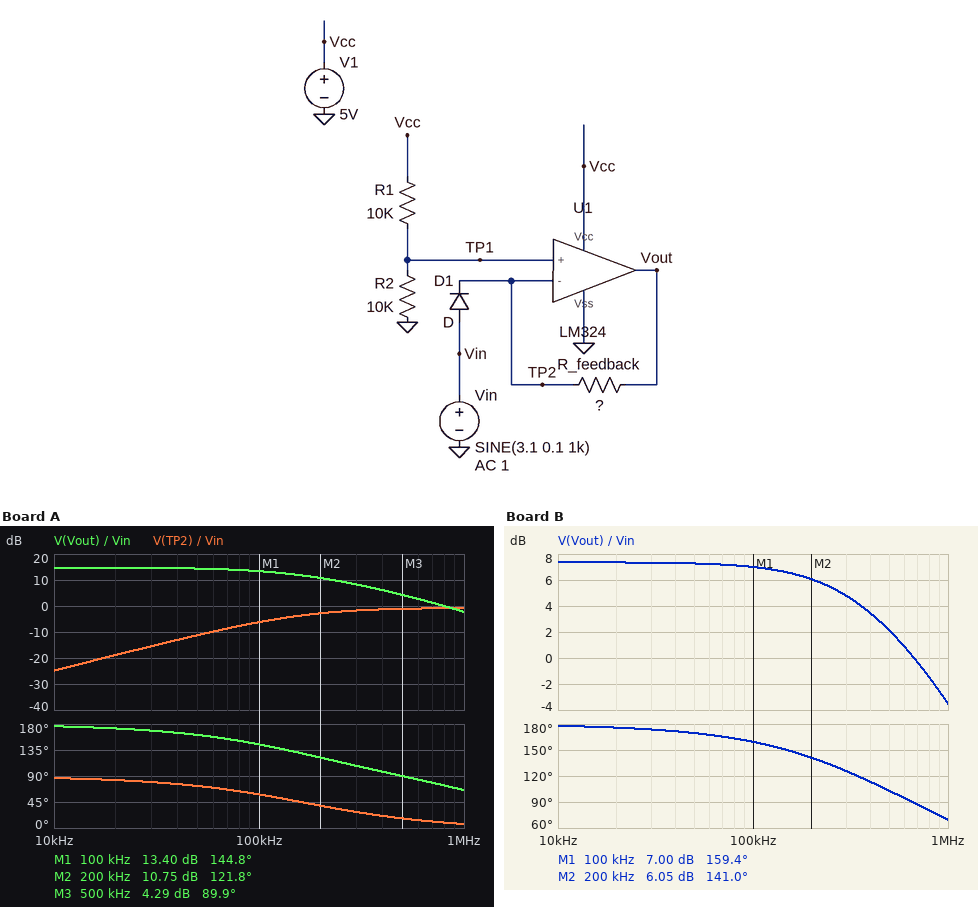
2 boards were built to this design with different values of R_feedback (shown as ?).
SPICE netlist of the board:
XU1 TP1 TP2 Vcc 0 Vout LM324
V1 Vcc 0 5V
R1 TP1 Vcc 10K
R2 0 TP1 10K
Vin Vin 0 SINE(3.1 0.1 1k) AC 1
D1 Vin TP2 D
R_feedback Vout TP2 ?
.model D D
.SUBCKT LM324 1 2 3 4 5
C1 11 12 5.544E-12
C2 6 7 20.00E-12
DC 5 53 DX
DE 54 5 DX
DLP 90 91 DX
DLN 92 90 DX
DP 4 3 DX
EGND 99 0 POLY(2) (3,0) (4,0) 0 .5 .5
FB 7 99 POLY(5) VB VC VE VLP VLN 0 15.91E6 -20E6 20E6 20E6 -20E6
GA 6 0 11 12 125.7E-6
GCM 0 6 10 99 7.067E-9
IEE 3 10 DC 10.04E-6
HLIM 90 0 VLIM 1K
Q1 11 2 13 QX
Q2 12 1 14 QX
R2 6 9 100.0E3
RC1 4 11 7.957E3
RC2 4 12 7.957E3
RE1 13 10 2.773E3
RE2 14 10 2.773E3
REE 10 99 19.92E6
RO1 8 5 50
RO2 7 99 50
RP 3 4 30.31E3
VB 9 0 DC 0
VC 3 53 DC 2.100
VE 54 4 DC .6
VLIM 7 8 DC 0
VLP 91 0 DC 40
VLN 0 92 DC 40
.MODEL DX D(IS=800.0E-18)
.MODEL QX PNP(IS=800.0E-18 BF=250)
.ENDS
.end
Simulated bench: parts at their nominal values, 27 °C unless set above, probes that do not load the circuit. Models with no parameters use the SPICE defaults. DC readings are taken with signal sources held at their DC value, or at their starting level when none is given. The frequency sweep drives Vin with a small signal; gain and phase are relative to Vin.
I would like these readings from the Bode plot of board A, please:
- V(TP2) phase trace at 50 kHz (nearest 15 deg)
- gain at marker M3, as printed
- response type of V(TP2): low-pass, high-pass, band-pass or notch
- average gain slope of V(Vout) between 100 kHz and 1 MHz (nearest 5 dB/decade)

75 deg
4.29 dB
high-pass
-15 dB/decade
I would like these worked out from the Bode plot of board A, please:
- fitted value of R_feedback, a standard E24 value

1.2 kΩ
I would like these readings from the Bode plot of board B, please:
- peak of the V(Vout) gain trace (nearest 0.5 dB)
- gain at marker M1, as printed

7.5 dB
7.00 dB
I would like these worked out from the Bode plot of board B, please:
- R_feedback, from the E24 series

510 Ω
